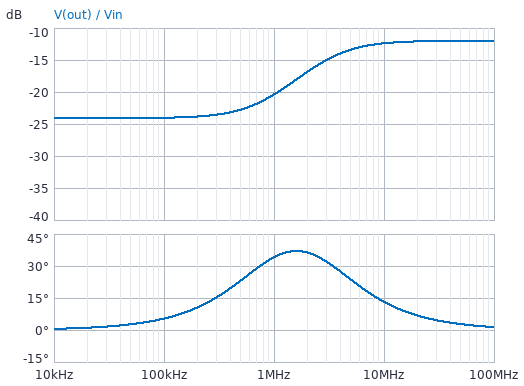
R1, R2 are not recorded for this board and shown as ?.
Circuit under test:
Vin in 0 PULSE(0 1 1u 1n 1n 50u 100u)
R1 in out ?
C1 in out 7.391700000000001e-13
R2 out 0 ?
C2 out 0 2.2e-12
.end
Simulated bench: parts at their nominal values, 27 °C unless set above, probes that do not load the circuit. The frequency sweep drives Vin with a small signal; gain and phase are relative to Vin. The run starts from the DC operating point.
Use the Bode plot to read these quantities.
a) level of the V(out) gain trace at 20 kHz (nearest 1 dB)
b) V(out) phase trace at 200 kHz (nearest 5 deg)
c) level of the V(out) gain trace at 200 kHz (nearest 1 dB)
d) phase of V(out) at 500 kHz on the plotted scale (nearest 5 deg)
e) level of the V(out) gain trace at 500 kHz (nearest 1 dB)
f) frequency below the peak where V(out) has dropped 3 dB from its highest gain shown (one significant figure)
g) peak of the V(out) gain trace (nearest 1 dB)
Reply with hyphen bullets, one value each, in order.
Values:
- -24 dB
- 10 deg
- -24 dB
- 25 deg
- -23 dB
- 3 MHz
- -12 dB
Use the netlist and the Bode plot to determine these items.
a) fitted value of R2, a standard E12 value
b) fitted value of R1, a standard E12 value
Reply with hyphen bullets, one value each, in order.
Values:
- 18 kΩ
- 270 kΩ
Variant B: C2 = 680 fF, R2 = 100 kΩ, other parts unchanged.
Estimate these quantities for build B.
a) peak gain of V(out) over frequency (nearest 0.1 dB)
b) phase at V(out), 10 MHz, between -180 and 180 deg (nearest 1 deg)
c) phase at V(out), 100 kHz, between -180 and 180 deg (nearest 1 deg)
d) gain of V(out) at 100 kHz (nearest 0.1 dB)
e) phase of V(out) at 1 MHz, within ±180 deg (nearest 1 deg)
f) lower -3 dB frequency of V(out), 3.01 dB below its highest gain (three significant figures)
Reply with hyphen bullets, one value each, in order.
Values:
- -5.7 dB
- 4 deg
- 3 deg
- -11.3 dB
- 18 deg
- 1.04 MHz
